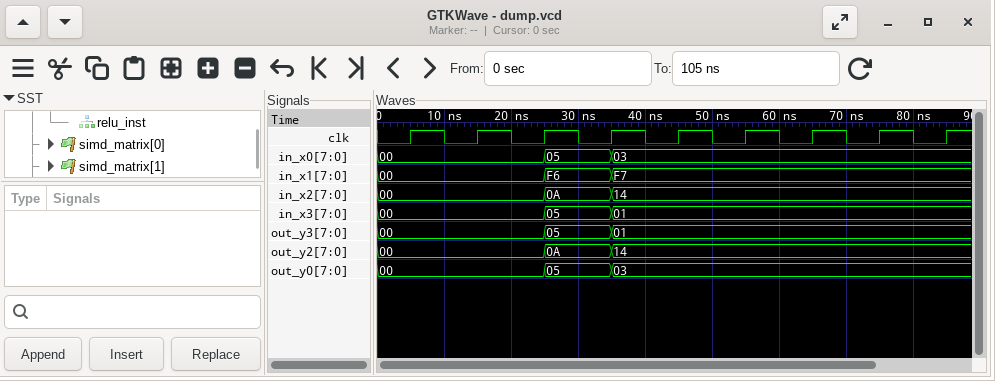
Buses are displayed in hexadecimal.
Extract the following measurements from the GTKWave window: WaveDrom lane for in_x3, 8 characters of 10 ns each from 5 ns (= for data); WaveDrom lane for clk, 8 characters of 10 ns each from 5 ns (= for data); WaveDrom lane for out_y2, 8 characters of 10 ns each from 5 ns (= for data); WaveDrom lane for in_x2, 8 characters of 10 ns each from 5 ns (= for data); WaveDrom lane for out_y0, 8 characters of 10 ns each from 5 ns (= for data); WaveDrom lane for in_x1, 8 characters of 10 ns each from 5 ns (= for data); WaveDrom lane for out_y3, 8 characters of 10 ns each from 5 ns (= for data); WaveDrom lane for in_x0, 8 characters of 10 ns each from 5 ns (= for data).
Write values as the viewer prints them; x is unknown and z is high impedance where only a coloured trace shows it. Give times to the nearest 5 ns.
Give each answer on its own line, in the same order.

{name: 'in_x3', wave: '=.==....', data: '00 05 01'}
{name: 'clk', wave: 'p.......'}
{name: 'out_y2', wave: '=.==....', data: '00 0A 14'}
{name: 'in_x2', wave: '=.==....', data: '00 0A 14'}
{name: 'out_y0', wave: '=.==....', data: '00 05 03'}
{name: 'in_x1', wave: '=.==....', data: '00 F6 F7'}
{name: 'out_y3', wave: '=.==....', data: '00 05 01'}
{name: 'in_x0', wave: '=.==....', data: '00 05 03'}
